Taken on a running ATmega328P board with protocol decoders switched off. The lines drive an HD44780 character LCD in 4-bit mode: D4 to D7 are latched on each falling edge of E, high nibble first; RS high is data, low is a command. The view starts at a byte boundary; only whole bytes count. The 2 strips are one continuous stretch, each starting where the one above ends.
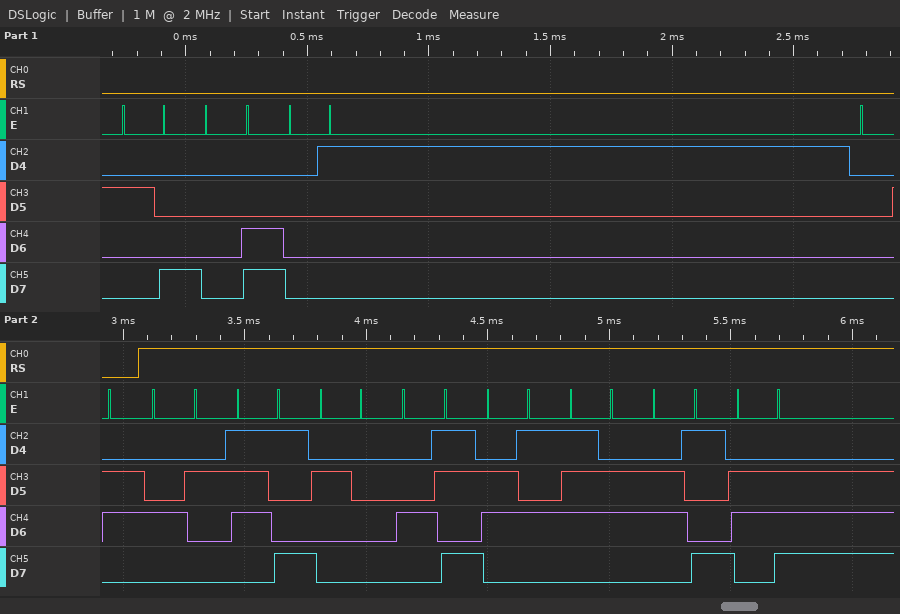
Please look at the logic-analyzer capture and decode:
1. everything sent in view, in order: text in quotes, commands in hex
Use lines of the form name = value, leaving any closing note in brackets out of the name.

everything sent in view, in order: text in quotes, commands in hex = 0x28 0x0C 0x01 0x06 "By Kevin"
